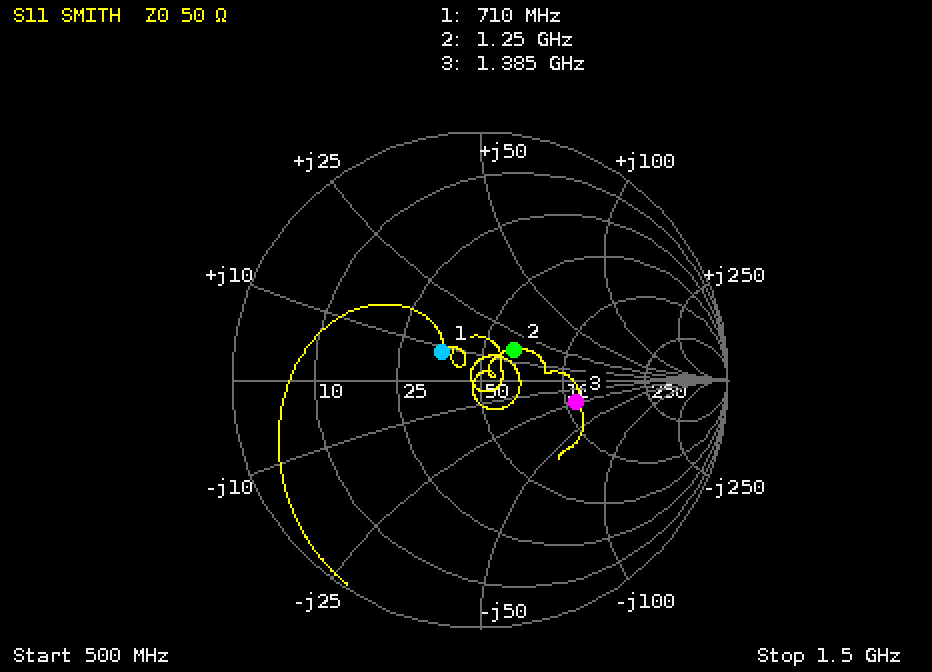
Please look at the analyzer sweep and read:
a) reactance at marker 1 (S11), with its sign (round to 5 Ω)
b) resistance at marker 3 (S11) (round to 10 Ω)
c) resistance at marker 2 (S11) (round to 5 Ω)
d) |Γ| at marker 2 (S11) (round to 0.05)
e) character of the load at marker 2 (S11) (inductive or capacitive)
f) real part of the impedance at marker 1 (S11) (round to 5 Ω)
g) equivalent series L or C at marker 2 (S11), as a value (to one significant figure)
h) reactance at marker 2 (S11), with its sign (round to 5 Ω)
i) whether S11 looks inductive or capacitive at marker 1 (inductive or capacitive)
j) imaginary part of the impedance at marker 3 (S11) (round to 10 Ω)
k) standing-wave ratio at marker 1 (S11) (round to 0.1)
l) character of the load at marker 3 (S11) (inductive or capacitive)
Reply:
+10 Ω
110 Ω
65 Ω
0.20
inductive
35 Ω
2 nH
+15 Ω
inductive
-20 Ω
1.5
capacitive
